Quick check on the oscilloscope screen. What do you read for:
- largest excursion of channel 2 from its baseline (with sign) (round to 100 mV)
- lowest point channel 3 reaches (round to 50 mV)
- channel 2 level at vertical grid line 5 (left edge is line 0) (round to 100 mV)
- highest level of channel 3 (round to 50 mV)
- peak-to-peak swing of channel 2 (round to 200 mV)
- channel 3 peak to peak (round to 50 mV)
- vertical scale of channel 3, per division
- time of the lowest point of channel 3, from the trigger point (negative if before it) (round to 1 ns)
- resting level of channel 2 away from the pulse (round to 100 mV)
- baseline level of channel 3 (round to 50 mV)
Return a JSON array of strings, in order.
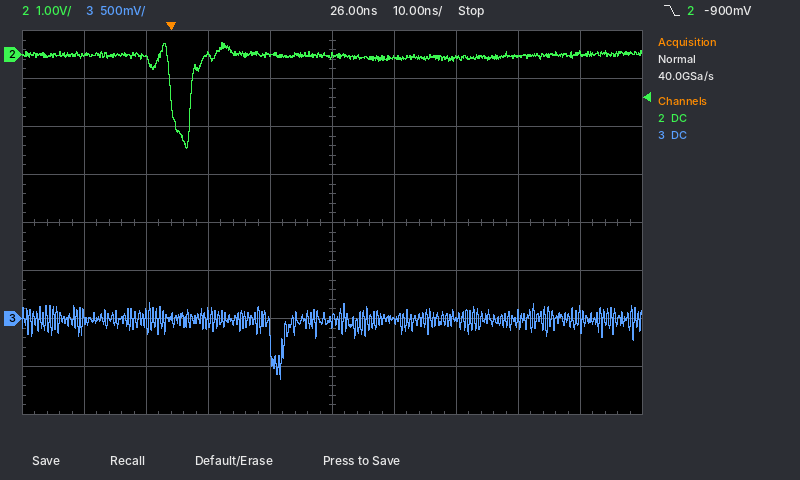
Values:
["-1.9 V", "-650 mV", "0.0 V", "150 mV", "2.2 V", "800 mV", "500 mV", "+18 ns", "0.0 V", "0 mV"]
